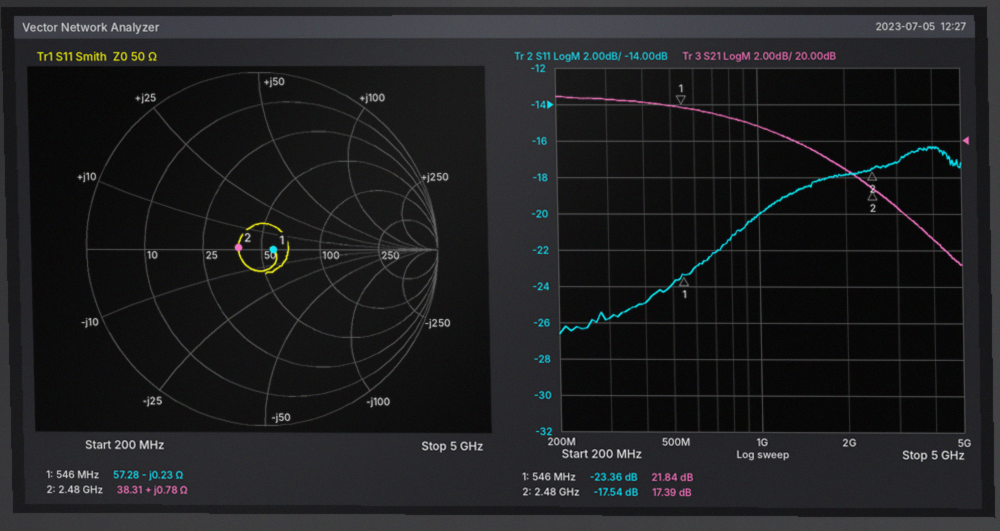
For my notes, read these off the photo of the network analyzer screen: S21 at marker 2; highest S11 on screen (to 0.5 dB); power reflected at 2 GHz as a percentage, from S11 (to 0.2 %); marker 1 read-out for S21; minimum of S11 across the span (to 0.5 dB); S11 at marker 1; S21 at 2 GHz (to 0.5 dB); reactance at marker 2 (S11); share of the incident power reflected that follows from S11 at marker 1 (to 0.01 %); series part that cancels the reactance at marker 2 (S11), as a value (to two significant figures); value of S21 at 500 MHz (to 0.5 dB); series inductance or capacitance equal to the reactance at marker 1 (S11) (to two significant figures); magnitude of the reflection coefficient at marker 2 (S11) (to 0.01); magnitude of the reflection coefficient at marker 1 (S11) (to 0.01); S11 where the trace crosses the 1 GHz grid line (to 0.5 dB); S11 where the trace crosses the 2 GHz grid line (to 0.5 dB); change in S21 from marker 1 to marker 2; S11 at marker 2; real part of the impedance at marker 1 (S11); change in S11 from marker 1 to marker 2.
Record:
17.39 dB
-16.5 dB
1.6 %
21.84 dB
-26.5 dB
-23.36 dB
18.5 dB
+0.78 Ω
0.46 %
82 pF
22.0 dB
1.3 nF
0.13
0.07
-20.0 dB
-18.0 dB
-4.45 dB
-17.54 dB
57.28 Ω
5.82 dB
